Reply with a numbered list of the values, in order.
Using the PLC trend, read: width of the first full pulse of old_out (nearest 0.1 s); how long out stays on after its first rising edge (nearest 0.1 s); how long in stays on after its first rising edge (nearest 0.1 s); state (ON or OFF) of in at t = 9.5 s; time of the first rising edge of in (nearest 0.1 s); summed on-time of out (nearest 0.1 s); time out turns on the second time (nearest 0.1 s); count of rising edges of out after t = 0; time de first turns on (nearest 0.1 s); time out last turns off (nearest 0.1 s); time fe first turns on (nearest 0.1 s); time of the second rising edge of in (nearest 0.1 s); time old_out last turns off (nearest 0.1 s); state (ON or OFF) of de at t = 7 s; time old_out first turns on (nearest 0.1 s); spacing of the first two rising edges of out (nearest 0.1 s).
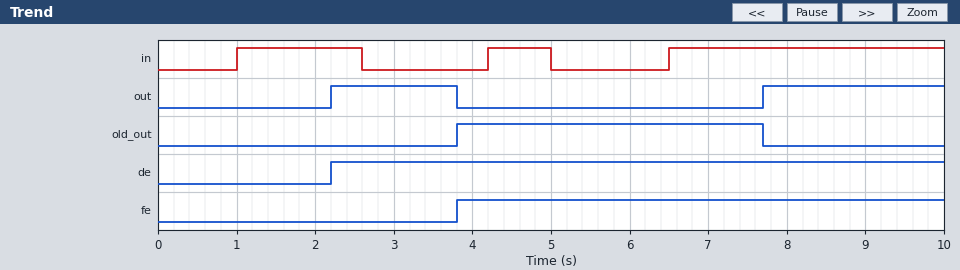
1. 3.9 s
2. 1.6 s
3. 1.6 s
4. ON
5. 1.0 s
6. 3.9 s
7. 7.7 s
8. 2
9. 2.2 s
10. 3.8 s
11. 3.8 s
12. 4.2 s
13. 7.7 s
14. ON
15. 3.8 s
16. 5.5 s
